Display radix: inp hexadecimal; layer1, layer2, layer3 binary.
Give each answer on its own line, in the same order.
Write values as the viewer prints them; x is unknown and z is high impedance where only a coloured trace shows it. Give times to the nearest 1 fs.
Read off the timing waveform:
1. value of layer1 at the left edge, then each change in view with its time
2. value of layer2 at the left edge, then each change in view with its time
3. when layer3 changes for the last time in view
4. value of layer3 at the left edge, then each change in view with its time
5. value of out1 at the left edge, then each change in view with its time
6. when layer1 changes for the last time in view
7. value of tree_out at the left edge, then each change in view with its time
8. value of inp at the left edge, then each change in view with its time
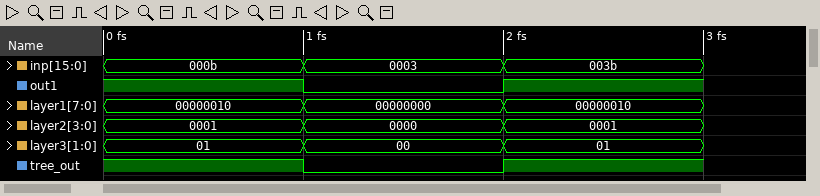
00000010, 00000000 at 1 fs, 00000010 at 2 fs
0001, 0000 at 1 fs, 0001 at 2 fs
2 fs
01, 00 at 1 fs, 01 at 2 fs
1, 0 at 1 fs, 1 at 2 fs
2 fs
1, 0 at 1 fs, 1 at 2 fs
000b, 0003 at 1 fs, 003b at 2 fs
